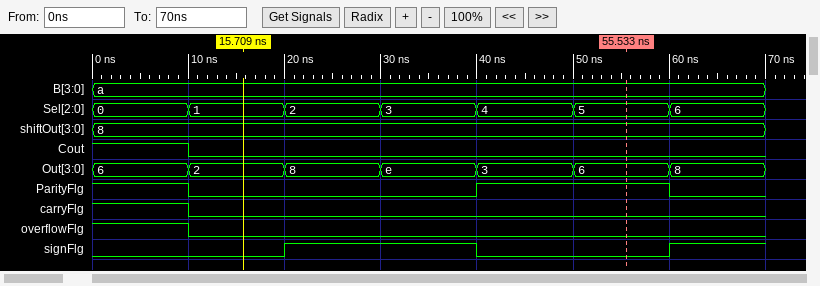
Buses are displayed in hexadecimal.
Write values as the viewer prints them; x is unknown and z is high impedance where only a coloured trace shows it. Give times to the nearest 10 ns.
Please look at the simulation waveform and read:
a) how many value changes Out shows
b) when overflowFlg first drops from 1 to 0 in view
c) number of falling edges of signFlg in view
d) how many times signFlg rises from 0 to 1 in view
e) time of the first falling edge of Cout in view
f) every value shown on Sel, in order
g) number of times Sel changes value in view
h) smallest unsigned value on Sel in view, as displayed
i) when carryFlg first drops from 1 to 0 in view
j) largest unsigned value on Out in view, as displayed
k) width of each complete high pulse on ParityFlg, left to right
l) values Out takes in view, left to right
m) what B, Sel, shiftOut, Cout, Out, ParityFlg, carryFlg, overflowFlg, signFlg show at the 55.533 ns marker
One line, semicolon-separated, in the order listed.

6; 10 ns; 1; 2; 10 ns; 0, 1, 2, 3, 4, 5, 6; 6; 0; 10 ns; e; 20 ns; 6, 2, 8, e, 3, 6, 8; B=a, Sel=5, shiftOut=8, Cout=0, Out=6, ParityFlg=1, carryFlg=0, overflowFlg=0, signFlg=0
